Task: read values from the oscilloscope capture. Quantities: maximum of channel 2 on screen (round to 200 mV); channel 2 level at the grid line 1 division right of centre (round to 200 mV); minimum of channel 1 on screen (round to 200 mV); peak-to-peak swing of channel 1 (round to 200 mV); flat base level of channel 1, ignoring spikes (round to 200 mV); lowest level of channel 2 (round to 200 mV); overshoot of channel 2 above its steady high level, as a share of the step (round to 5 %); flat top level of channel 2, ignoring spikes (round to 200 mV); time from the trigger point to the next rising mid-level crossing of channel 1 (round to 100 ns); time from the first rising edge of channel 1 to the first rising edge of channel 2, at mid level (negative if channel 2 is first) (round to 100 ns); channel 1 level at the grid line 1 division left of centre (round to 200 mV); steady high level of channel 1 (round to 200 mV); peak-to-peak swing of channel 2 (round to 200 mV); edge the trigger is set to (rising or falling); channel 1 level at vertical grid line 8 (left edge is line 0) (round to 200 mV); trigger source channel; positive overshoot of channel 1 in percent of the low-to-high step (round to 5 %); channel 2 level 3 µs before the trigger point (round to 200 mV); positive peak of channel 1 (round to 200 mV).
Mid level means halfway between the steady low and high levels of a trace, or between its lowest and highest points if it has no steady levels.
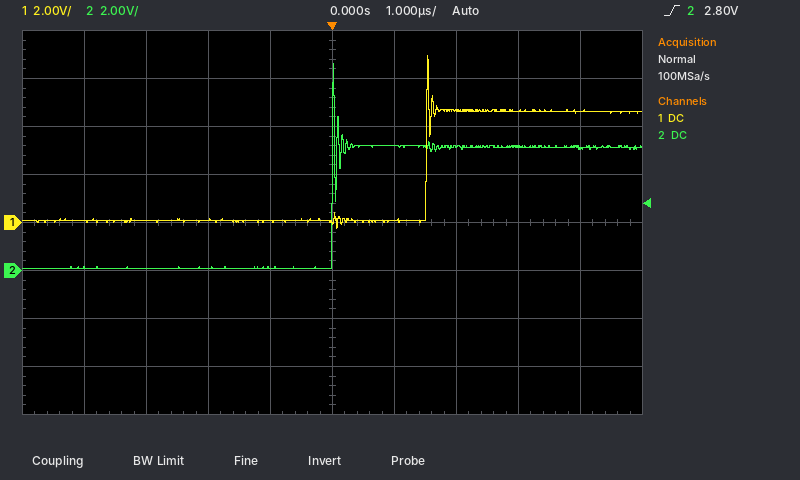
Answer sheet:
8.6 V
5.2 V
-200 mV
7.2 V
0.0 V
0.0 V
70 %
5.2 V
1.5 µs
-1.5 µs
0.0 V
4.6 V
8.6 V
rising
4.6 V
channel 2
50 %
0.0 V
7.0 V
